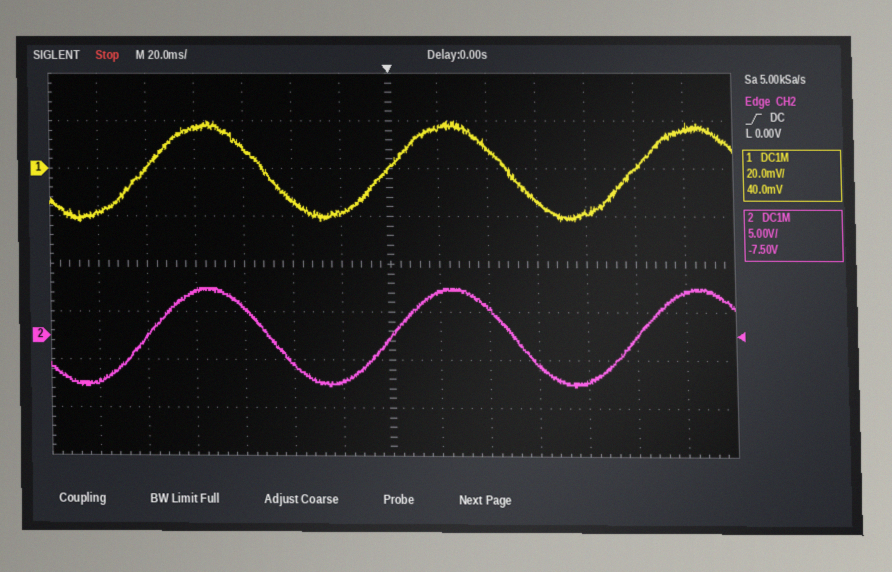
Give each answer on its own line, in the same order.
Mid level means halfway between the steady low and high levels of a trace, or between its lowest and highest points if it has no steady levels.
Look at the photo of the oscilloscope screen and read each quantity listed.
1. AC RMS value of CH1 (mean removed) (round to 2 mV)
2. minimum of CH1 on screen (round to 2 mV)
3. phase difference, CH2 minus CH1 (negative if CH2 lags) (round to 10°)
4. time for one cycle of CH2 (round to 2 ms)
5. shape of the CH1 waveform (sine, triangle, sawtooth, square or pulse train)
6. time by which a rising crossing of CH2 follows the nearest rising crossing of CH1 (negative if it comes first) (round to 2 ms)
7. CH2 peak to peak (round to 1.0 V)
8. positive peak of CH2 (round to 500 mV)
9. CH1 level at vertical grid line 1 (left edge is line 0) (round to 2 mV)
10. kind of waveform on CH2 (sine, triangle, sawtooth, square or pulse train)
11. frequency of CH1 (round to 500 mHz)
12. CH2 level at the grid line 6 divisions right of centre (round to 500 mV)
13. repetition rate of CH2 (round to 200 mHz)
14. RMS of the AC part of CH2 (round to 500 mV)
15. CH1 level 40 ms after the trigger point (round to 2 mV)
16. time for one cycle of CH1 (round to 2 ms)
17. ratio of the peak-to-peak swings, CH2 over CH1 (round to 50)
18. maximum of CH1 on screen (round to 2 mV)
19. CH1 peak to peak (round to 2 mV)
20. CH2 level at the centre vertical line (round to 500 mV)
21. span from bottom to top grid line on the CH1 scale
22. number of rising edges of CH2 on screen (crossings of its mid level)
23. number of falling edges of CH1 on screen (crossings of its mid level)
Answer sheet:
14 mV
-22 mV
0°
100 ms
sine
0 ms
10.0 V
5.0 V
-18 mV
sine
10.0 Hz
4.5 V
10.0 Hz
3.5 V
8 mV
100 ms
250
20 mV
42 mV
0.0 V
160 mV
3
2
